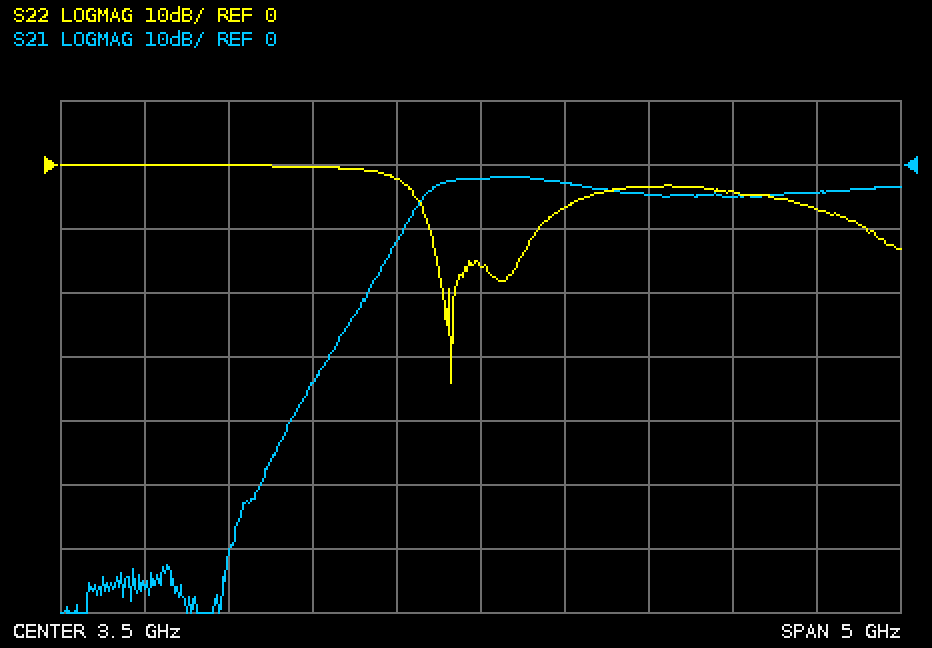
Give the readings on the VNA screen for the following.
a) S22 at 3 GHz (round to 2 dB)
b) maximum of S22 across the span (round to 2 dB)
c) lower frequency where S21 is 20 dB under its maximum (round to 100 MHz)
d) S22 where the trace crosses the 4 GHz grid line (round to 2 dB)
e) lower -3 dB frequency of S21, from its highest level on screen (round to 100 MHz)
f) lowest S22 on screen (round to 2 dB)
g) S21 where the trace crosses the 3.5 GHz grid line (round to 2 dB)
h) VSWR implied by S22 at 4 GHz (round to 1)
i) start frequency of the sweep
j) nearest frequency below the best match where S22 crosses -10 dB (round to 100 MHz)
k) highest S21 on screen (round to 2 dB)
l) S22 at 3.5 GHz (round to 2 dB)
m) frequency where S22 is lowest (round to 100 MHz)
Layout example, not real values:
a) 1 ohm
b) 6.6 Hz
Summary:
a) -2 dB
b) 0 dB
c) 2.8 GHz
d) -6 dB
e) 3.2 GHz
f) -34 dB
g) -2 dB
h) 3
i) 1 GHz
j) 3.2 GHz
k) -2 dB
l) -16 dB
m) 3.3 GHz
